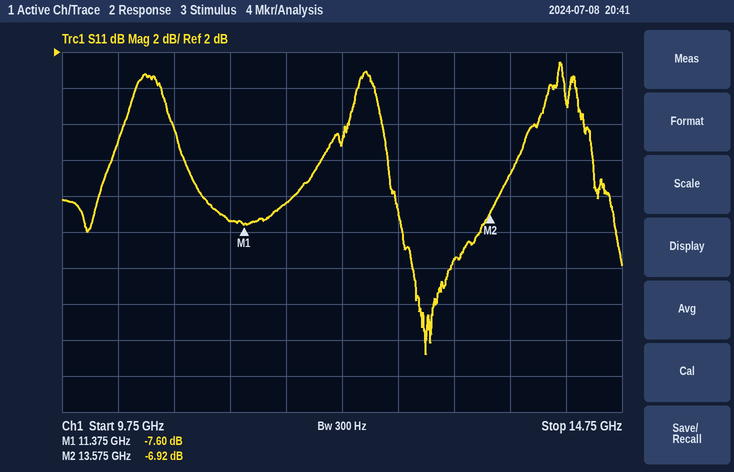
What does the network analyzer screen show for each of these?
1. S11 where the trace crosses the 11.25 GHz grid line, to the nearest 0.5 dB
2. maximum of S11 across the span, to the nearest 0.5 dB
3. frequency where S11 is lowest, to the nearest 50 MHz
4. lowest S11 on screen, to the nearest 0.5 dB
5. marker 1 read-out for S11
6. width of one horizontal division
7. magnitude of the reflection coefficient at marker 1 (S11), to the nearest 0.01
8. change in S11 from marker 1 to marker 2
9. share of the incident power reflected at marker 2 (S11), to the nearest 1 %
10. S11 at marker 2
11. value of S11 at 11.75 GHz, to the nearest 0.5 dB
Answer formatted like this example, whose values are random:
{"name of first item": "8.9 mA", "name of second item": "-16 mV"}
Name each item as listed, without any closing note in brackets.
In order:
{"S11 where the trace crosses the 11.25 GHz grid line, to the nearest 0.5 dB": "-7.5 dB", "maximum of S11 across the span, to the nearest 0.5 dB": "1.5 dB", "frequency where S11 is lowest, to the nearest 50 MHz": "13.00 GHz", "lowest S11 on screen, to the nearest 0.5 dB": "-15.0 dB", "marker 1 read-out for S11": "-7.60 dB", "width of one horizontal division": "500 MHz", "magnitude of the reflection coefficient at marker 1 (S11), to the nearest 0.01": "0.42", "change in S11 from marker 1 to marker 2": "0.68 dB", "share of the incident power reflected at marker 2 (S11), to the nearest 1 %": "20 %", "S11 at marker 2": "-6.92 dB", "value of S11 at 11.75 GHz, to the nearest 0.5 dB": "-6.5 dB"}
